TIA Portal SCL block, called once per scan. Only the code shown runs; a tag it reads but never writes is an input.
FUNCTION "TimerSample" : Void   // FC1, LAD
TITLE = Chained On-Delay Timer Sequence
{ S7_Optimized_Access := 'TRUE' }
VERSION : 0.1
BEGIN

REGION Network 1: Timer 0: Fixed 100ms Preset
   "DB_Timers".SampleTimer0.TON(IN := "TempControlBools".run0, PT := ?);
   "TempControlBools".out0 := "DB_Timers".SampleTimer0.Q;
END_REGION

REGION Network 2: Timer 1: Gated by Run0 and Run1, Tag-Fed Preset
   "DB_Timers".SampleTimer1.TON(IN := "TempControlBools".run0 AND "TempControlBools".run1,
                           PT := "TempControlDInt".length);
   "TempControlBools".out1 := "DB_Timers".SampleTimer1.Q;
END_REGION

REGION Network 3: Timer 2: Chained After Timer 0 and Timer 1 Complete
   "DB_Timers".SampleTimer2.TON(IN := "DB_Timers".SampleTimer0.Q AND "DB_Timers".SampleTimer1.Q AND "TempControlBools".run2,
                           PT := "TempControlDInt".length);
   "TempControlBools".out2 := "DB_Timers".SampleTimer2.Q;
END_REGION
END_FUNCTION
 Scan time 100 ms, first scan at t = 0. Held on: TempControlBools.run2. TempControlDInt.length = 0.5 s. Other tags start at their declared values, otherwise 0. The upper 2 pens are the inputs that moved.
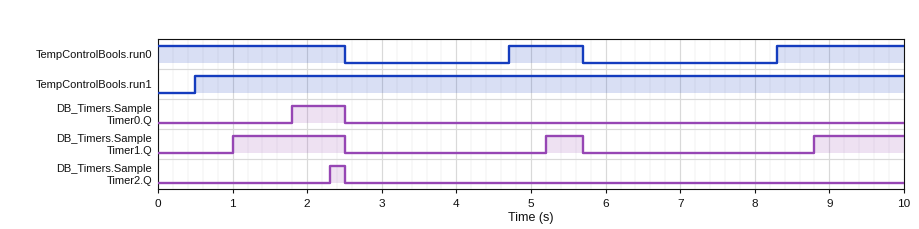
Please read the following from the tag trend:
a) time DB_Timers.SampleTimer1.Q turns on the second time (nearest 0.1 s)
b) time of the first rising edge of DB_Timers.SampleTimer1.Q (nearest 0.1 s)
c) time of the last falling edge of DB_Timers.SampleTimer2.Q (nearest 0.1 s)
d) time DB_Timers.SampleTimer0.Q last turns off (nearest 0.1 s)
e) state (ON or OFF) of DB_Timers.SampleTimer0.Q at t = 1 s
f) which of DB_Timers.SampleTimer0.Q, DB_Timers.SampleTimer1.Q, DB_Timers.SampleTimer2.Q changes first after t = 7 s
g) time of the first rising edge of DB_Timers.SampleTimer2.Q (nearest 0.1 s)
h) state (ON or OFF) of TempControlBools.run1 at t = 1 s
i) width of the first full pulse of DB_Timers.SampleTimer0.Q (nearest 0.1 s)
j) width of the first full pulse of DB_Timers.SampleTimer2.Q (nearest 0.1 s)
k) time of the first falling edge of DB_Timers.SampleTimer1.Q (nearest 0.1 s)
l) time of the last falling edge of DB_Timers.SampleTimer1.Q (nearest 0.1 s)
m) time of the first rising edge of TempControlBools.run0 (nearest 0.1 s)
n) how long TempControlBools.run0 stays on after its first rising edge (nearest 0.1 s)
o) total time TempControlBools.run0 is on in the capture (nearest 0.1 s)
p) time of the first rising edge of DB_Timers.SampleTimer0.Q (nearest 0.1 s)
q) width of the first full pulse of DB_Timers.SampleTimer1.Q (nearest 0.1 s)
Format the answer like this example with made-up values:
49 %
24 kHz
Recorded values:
5.2 s
1.0 s
2.5 s
2.5 s
OFF
DB_Timers.SampleTimer1.Q
2.3 s
ON
0.7 s
0.2 s
2.5 s
5.7 s
4.7 s
1.0 s
5.2 s
1.8 s
1.5 s
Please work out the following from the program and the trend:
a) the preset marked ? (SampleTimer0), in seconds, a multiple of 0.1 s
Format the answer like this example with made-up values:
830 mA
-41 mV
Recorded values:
1.8 s
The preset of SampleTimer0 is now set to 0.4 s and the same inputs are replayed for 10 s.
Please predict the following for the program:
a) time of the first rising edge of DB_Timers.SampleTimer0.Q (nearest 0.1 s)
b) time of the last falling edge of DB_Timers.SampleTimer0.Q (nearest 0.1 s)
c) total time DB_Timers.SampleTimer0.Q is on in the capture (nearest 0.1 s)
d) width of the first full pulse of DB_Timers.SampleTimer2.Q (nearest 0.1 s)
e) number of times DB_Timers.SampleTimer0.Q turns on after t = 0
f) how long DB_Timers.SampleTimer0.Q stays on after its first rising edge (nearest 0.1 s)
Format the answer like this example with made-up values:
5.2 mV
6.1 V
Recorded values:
0.4 s
5.7 s
4.0 s
1.0 s
3
2.1 s
